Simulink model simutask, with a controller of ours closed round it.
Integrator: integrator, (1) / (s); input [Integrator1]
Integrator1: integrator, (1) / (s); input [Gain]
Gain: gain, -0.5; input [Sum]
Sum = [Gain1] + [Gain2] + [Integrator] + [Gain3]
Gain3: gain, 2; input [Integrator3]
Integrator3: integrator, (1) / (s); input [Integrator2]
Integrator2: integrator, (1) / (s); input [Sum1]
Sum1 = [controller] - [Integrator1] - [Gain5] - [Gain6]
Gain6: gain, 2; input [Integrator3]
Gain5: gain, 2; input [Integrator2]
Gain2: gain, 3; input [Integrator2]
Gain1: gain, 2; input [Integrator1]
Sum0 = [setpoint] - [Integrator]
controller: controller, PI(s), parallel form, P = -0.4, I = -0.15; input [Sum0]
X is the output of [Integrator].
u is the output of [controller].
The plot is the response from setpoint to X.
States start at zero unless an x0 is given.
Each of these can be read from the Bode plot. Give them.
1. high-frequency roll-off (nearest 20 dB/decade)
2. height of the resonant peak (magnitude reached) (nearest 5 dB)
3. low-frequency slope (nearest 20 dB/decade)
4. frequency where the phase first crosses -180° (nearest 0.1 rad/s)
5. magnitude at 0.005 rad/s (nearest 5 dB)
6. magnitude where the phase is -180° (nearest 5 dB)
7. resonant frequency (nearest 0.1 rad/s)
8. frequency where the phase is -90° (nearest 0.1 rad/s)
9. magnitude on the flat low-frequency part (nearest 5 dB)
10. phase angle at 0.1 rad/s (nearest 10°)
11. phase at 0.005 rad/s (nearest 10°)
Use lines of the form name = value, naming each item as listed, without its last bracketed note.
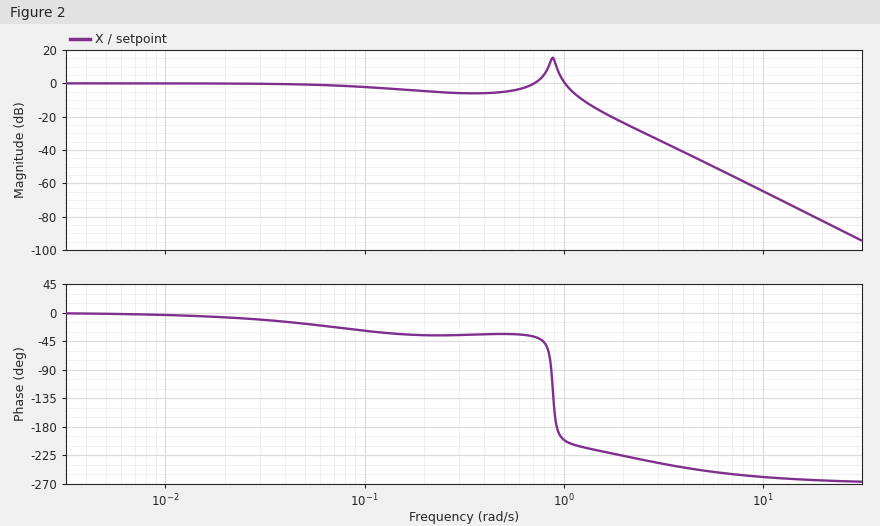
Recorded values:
high-frequency roll-off = -60 dB/decade
height of the resonant peak (magnitude reached) = 15 dB
low-frequency slope = 0 dB/decade
frequency where the phase first crosses -180° = 0.9 rad/s
magnitude at 0.005 rad/s = 0 dB
magnitude where the phase is -180° = 10 dB
resonant frequency = 0.9 rad/s
frequency where the phase is -90° = 0.9 rad/s
magnitude on the flat low-frequency part = 0 dB
phase angle at 0.1 rad/s = -30°
phase at 0.005 rad/s = 0°
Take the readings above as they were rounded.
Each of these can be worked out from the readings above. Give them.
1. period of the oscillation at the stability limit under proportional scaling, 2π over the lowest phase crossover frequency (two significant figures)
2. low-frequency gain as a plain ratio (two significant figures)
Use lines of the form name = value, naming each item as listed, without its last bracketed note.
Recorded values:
period of the oscillation at the stability limit under proportional scaling, 2π over the lowest phase crossover frequency = 7.0 s
low-frequency gain as a plain ratio = 1.0
